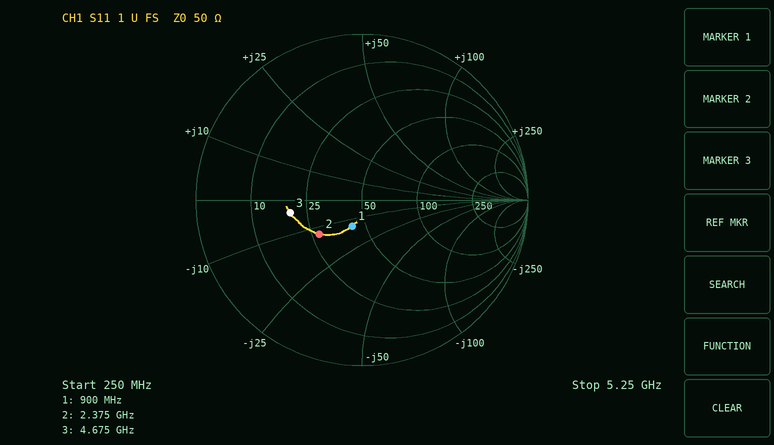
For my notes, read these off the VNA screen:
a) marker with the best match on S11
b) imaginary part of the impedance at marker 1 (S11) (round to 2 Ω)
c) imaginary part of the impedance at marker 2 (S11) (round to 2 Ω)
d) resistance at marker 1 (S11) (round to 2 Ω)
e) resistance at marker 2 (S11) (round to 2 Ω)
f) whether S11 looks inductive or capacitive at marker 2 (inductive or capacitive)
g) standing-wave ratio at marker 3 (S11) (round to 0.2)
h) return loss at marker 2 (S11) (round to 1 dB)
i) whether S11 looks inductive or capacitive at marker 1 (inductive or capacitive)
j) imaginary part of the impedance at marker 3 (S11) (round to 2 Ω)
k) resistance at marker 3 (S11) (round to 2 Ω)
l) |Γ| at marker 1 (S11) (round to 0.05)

marker 1
-14 Ω
-12 Ω
42 Ω
28 Ω
capacitive
2.6
10 dB
capacitive
-4 Ω
20 Ω
0.15
